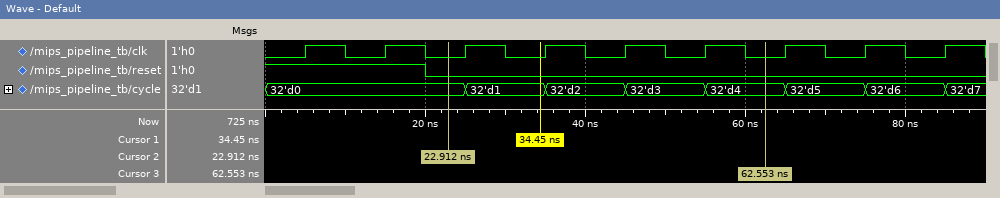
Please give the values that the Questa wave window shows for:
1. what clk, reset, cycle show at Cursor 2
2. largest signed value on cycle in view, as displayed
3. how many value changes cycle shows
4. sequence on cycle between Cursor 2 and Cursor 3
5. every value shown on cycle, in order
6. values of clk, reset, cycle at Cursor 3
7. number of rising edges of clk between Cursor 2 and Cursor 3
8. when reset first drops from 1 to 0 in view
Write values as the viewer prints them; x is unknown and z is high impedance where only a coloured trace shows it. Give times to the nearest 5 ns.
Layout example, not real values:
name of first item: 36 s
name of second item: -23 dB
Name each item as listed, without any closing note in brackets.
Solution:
what clk, reset, cycle show at Cursor 2: clk=0, reset=0, cycle=32'd0
largest signed value on cycle in view, as displayed: 32'd7
how many value changes cycle shows: 7
sequence on cycle between Cursor 2 and Cursor 3: 32'd0, 32'd1, 32'd2, 32'd3, 32'd4
every value shown on cycle, in order: 32'd0, 32'd1, 32'd2, 32'd3, 32'd4, 32'd5, 32'd6, 32'd7
values of clk, reset, cycle at Cursor 3: clk=0, reset=0, cycle=32'd4
number of rising edges of clk between Cursor 2 and Cursor 3: 4
when reset first drops from 1 to 0 in view: 20 ns
